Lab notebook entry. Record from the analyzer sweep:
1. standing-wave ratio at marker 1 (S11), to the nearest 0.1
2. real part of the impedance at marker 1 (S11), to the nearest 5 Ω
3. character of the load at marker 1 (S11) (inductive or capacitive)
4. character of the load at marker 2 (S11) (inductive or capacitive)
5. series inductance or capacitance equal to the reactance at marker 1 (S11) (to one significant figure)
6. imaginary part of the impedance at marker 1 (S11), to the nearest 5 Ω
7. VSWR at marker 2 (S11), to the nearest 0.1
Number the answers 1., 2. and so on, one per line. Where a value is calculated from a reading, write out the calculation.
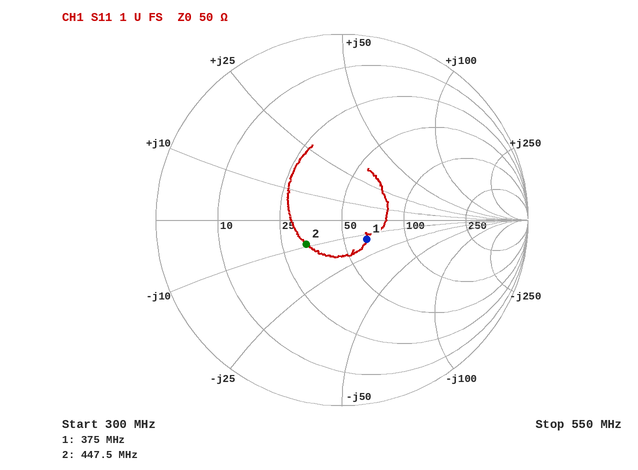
1. 1.4
2. 65 Ω
3. capacitive
4. capacitive
5. C = 1/(2π × 375 MHz × 15 Ω) ≈ 28.3 pF, so 30 pF to one significant figure
6. -15 Ω
7. 1.6
